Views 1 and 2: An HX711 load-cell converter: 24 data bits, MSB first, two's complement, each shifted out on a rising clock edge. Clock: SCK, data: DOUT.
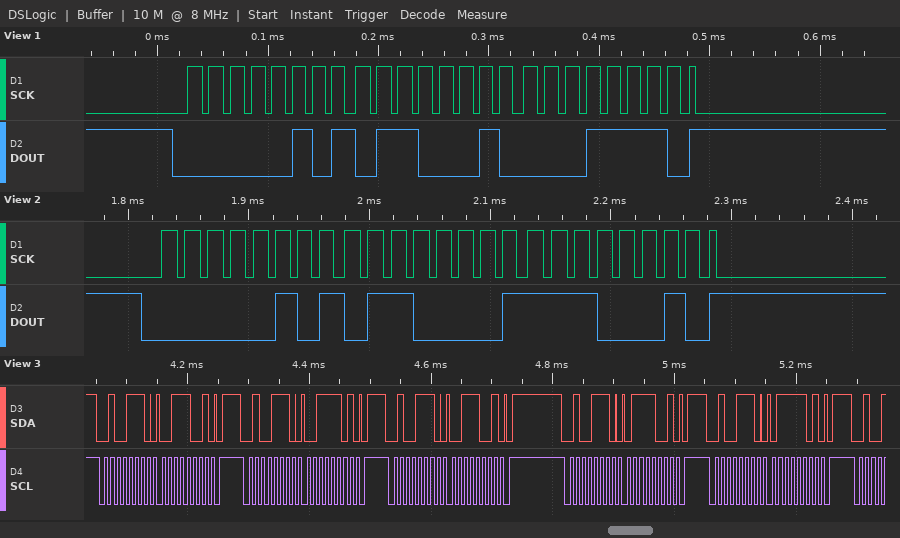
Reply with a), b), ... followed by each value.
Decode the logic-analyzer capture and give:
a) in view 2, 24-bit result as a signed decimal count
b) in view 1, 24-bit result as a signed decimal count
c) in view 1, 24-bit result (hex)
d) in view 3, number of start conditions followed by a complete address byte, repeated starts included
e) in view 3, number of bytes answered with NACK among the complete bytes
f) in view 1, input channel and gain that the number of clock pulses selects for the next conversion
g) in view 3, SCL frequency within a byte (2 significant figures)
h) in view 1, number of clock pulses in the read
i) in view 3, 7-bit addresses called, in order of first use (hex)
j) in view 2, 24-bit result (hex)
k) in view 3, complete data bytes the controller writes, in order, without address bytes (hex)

a) 352738
b) 352798
c) 0x05621E
d) 5
e) 0
f) channel A, gain 128
g) 100 kHz
h) 25
i) 0x27
j) 0x0561E2
k) 39 3D 39 79 7D
